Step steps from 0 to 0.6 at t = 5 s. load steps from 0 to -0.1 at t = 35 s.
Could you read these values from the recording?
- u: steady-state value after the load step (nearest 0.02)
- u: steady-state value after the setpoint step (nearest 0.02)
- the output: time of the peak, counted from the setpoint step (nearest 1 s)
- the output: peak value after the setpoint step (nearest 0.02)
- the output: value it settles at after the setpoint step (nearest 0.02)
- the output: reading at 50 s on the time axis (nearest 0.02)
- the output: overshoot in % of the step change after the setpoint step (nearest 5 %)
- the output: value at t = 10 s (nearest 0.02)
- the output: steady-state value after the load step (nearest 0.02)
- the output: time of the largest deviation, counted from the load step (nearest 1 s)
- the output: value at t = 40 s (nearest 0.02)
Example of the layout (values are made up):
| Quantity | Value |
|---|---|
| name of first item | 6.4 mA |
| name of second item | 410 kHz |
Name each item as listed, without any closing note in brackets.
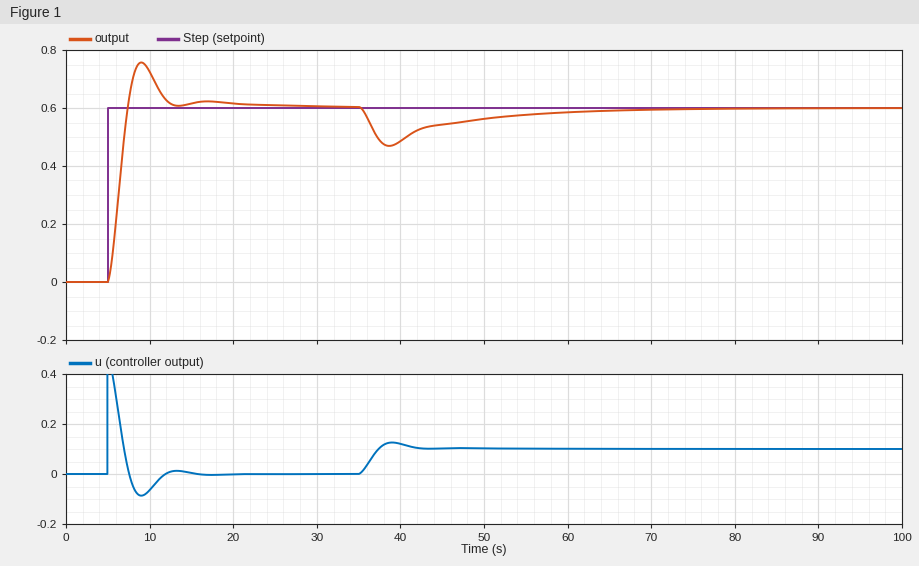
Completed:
| Quantity | Value |
|---|---|
| u: steady-state value after the load step | 0.10 |
| u: steady-state value after the setpoint step | 0.00 |
| the output: time of the peak, counted from the setpoint step | 4 s |
| the output: peak value after the setpoint step | 0.76 |
| the output: value it settles at after the setpoint step | 0.60 |
| the output: reading at 50 s on the time axis | 0.56 |
| the output: overshoot in % of the step change after the setpoint step | 25 % |
| the output: value at t = 10 s | 0.72 |
| the output: steady-state value after the load step | 0.60 |
| the output: time of the largest deviation, counted from the load step | 4 s |
| the output: value at t = 40 s | 0.48 |
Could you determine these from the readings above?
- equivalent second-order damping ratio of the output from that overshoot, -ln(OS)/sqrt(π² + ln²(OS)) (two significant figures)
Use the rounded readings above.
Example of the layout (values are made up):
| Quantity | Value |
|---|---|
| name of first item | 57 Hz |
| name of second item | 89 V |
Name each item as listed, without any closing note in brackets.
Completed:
| Quantity | Value |
|---|---|
| equivalent second-order damping ratio of the output from that overshoot, -ln(OS)/sqrt(π² + ln²(OS)) | 0.40 |
